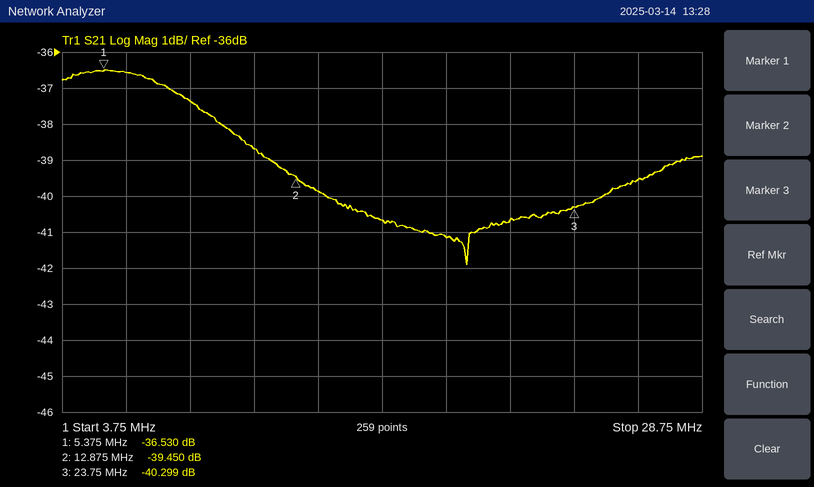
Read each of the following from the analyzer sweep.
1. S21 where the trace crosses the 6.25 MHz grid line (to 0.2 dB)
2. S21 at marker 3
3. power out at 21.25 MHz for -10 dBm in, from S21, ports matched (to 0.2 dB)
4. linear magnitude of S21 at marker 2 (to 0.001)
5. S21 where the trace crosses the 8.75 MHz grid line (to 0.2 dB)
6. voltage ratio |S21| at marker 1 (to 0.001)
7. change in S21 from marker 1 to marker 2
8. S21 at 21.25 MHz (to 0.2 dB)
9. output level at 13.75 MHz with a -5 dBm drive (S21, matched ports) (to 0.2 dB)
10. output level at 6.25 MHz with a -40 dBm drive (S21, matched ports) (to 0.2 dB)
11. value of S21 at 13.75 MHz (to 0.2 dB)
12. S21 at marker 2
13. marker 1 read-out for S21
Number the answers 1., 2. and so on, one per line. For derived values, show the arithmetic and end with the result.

1. -36.6 dB
2. -40.299 dB
3. -10 dBm + (-40.6 dB) = -50.6 dBm
4. 10^(-39.45/20) ≈ 0.011
5. -37.4 dB
6. 10^(-36.53/20) ≈ 0.015
7. -39.45 − (-36.53) = -2.920 dB
8. -40.6 dB
9. -5 dBm + (-39.8 dB) = -44.8 dBm
10. -40 dBm + (-36.6 dB) = -76.6 dBm
11. -39.8 dB
12. -39.450 dB
13. -36.530 dB
